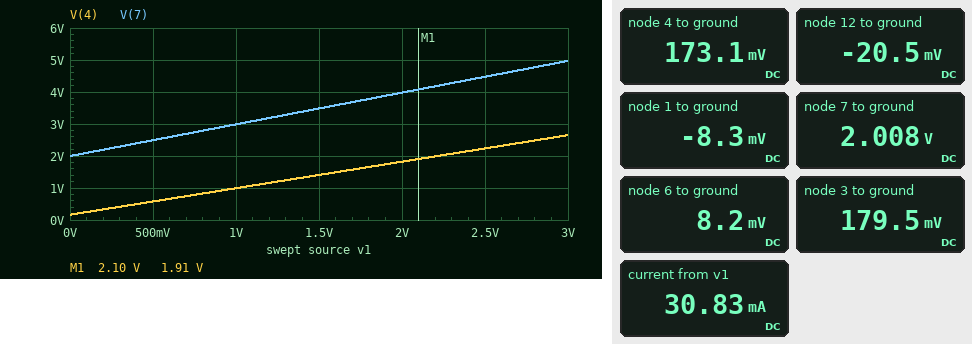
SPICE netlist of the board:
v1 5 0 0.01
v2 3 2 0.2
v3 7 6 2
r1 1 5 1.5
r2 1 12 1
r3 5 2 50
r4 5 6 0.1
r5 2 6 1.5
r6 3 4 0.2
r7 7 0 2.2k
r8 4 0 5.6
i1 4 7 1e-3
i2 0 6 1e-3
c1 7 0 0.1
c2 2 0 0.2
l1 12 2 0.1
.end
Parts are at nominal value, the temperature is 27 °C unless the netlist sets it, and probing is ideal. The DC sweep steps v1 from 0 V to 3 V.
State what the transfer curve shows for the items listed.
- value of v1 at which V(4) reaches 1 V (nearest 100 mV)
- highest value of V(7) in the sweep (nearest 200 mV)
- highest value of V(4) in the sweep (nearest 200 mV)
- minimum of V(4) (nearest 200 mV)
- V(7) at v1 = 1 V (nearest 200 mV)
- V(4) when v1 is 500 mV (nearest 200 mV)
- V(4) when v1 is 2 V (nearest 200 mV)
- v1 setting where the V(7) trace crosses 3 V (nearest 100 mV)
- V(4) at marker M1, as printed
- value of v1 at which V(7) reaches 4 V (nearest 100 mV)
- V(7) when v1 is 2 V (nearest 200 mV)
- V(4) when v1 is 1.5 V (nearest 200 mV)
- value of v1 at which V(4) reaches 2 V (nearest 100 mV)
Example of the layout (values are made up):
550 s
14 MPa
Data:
1.0 V
5.0 V
2.6 V
200 mV
3.0 V
600 mV
1.8 V
1.0 V
1.91 V
2.0 V
4.0 V
1.4 V
2.2 V
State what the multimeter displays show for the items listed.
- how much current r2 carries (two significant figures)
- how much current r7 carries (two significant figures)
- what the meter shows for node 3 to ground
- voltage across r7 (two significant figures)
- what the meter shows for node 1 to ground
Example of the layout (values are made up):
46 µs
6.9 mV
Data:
12 mA
910 µA
179.5 mV
2.0 V
-8.3 mV
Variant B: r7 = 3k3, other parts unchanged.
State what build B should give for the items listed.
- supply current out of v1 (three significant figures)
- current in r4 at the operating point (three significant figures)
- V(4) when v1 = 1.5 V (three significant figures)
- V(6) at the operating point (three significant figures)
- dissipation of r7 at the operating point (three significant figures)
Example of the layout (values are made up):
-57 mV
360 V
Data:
30.5 mA
17.7 mA
1.41 V
8.23 mV
1.22 mW
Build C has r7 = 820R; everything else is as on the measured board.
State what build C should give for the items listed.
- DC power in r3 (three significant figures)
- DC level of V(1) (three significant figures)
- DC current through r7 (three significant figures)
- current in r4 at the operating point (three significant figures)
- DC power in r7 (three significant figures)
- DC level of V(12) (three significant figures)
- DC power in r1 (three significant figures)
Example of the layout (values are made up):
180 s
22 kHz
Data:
18.7 µW
-8.33 mV
2.45 mA
19.5 mA
4.92 mW
-20.6 mV
224 µW
